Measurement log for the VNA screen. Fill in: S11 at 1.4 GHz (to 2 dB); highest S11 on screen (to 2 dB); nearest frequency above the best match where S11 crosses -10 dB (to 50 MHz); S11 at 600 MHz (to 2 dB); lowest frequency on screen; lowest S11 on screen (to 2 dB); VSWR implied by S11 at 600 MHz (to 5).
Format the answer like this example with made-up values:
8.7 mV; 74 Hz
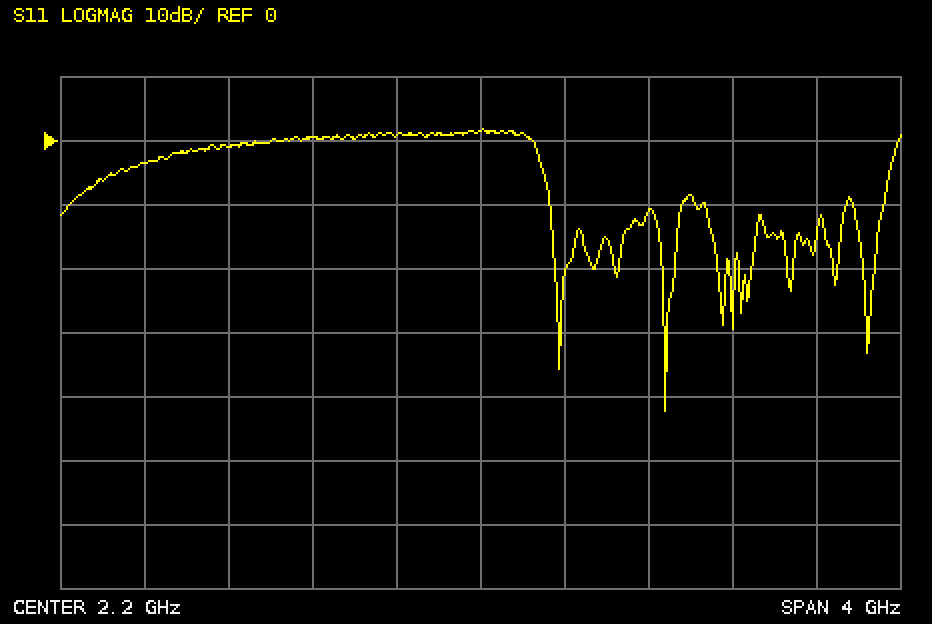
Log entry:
0 dB; 2 dB; 3.15 GHz; -4 dB; 200 MHz; -42 dB; 5
